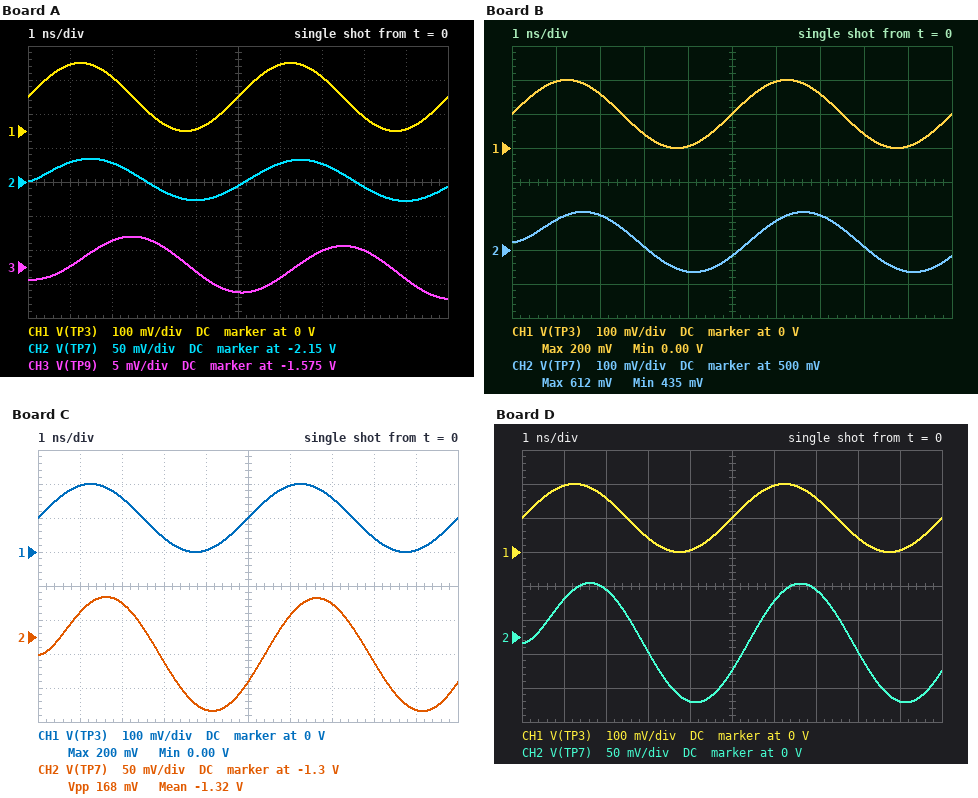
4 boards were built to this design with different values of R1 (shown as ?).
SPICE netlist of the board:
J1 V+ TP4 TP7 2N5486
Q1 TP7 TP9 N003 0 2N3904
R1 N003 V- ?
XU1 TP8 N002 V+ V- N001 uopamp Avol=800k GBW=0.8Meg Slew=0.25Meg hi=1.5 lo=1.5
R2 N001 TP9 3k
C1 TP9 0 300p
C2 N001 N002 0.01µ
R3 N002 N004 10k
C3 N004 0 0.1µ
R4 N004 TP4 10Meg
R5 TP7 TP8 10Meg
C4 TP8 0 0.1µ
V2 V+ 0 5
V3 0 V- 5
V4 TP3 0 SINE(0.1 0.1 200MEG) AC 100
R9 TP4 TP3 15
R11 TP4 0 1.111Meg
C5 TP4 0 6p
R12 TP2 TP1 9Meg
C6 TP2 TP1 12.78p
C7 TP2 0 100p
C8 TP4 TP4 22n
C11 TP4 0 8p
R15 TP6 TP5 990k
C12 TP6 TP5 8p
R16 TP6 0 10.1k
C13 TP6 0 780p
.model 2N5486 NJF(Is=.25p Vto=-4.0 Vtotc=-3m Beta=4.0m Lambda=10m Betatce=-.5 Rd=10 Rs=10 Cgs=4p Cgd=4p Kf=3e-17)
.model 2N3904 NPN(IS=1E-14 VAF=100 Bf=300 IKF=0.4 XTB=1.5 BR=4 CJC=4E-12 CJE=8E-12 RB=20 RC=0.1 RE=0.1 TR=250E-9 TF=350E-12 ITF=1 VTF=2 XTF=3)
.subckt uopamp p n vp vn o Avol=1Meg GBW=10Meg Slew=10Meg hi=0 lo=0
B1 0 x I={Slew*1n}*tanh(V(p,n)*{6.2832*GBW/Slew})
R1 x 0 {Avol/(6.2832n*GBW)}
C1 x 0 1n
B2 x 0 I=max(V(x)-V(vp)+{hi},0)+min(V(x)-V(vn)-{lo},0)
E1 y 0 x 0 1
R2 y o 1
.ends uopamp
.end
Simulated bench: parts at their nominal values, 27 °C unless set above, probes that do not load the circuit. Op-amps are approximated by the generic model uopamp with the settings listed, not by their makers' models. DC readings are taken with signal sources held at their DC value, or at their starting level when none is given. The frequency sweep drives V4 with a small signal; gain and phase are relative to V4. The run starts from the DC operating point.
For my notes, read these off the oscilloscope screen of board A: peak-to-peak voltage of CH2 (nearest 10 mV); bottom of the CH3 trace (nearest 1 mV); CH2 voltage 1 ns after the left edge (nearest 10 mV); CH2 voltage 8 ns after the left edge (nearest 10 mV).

60 mV
-1.580 V
-2.12 V
-2.16 V
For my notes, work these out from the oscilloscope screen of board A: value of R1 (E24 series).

22 Ω
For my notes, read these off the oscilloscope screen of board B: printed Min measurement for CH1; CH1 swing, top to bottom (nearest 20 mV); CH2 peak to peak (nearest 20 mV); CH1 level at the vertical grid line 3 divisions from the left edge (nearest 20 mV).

0.00 V
200 mV
180 mV
40 mV
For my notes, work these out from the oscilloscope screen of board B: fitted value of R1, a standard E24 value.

91 Ω
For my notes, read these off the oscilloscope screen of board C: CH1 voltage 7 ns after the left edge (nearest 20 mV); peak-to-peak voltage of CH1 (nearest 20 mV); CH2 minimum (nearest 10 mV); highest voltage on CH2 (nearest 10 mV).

160 mV
200 mV
-1.41 V
-1.24 V
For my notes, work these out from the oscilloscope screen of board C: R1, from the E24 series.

36 Ω
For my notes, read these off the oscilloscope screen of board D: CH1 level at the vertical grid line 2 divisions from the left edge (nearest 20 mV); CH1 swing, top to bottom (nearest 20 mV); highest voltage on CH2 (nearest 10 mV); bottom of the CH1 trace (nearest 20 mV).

160 mV
200 mV
80 mV
0 V
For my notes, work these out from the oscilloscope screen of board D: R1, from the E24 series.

68 Ω
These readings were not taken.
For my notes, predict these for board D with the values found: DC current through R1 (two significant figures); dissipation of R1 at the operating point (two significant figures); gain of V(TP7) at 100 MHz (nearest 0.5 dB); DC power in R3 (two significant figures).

52 mA
180 mW
-0.5 dB
980 nW
